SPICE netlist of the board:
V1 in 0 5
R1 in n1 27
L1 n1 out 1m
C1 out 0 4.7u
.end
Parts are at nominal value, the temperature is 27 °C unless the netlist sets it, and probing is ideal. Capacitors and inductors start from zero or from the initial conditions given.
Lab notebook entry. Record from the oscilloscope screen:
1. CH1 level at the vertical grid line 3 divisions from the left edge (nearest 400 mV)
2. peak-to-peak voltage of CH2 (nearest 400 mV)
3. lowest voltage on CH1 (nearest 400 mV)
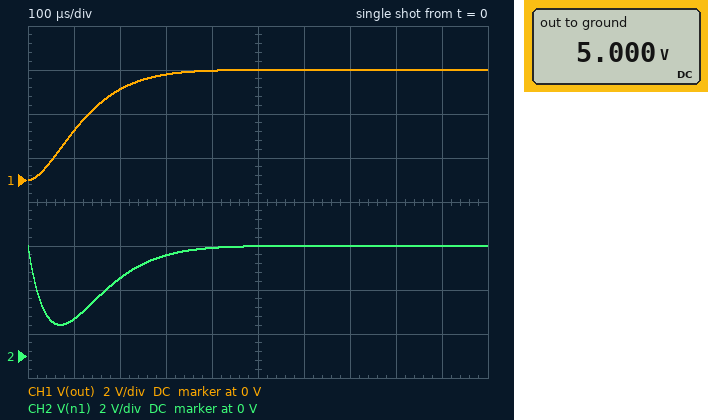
4.8 V
3.6 V
0 V
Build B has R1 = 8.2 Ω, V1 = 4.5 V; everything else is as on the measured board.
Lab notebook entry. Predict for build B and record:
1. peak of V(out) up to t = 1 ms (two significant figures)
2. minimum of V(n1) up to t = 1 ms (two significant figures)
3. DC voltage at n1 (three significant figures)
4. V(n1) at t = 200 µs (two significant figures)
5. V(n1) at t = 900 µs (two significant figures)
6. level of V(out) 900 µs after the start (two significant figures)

6.3 V
2.8 V
4.50 V
4.1 V
4.5 V
4.4 V
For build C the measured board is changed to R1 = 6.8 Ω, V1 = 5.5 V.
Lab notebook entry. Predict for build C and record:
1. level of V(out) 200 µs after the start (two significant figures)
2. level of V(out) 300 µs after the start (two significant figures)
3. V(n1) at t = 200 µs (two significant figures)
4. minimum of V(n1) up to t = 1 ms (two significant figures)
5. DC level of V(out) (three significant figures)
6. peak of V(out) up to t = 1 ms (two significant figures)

8.0 V
6.8 V
5.1 V
3.6 V
5.50 V
8.1 V
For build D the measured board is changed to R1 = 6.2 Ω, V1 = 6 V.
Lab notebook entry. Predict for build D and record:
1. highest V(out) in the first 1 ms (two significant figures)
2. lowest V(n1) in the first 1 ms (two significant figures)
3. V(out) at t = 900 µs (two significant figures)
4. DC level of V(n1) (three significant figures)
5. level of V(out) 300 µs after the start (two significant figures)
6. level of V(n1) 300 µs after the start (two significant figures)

9.0 V
4.1 V
5.6 V
6.00 V
7.5 V
6.9 V
